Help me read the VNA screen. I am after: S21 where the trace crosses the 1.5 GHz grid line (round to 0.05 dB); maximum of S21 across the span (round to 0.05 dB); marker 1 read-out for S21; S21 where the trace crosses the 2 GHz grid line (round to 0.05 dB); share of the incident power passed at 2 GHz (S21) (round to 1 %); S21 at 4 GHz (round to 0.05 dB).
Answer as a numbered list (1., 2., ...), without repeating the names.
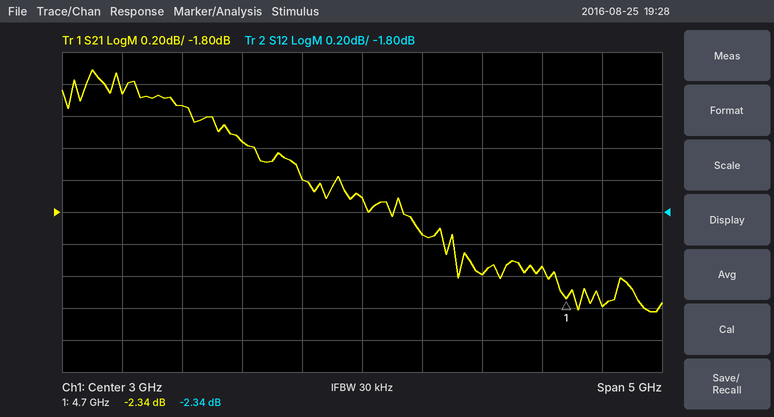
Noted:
1. -1.15 dB
2. -0.90 dB
3. -2.34 dB
4. -1.35 dB
5. 73 %
6. -2.20 dB
